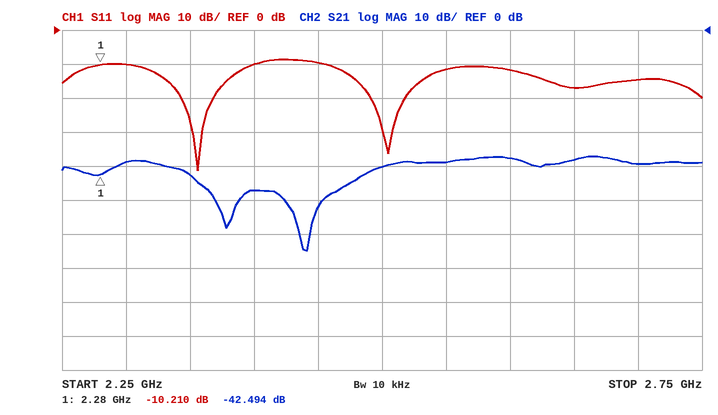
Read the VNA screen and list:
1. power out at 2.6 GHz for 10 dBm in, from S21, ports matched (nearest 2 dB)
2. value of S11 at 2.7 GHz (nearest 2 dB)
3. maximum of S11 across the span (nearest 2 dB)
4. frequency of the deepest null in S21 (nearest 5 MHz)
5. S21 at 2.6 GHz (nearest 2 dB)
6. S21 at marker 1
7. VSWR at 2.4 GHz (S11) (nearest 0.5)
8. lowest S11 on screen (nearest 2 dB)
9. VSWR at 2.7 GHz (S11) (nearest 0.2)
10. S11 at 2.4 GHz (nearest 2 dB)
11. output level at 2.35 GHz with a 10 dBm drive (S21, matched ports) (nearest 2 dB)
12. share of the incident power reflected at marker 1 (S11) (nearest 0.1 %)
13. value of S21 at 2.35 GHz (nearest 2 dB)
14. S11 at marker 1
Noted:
-28 dBm
-14 dB
-8 dB
2.440 GHz
-38 dB
-42.494 dB
2.0
-42 dB
1.4
-10 dB
-32 dBm
9.5 %
-42 dB
-10.210 dB
